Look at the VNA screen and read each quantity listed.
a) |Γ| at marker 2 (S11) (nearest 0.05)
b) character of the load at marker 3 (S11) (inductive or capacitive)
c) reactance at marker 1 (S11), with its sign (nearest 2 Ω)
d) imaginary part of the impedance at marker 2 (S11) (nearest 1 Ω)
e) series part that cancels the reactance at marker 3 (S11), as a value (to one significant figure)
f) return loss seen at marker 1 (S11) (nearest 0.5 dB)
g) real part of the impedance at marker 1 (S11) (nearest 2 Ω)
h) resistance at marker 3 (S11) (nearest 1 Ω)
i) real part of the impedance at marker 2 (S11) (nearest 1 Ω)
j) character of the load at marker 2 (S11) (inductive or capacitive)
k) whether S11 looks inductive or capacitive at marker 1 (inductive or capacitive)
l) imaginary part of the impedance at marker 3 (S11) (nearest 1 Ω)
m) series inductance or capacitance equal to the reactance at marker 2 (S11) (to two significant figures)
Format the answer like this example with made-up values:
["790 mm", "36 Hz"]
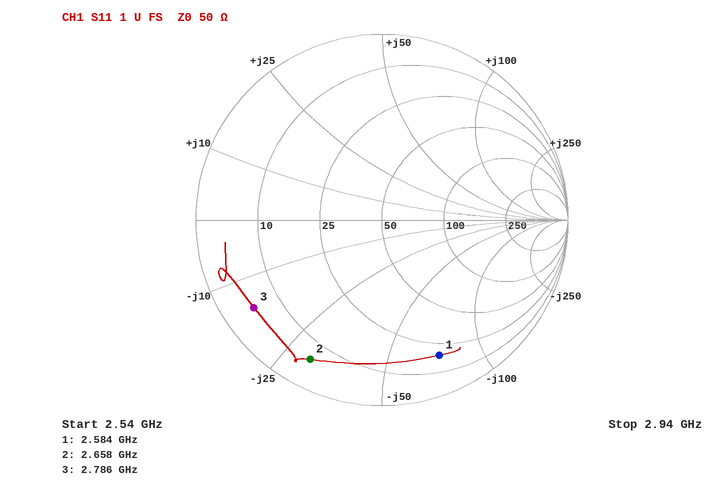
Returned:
["0.85", "capacitive", "-72 Ω", "-30 Ω", "900 pH", "2.0 dB", "18 Ω", "5 Ω", "6 Ω", "capacitive", "capacitive", "-15 Ω", "2.0 pF"]
